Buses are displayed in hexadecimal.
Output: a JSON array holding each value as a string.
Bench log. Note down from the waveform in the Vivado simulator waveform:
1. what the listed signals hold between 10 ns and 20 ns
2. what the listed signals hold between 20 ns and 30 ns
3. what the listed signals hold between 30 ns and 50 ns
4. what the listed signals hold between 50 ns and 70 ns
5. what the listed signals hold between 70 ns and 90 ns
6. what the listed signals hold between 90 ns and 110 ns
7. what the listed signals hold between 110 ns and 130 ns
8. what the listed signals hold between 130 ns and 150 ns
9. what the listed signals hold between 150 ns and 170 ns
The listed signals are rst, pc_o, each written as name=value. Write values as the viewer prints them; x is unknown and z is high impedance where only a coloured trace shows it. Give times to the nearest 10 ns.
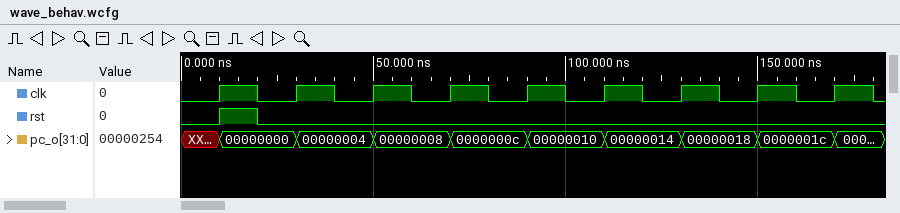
["rst=1, pc_o=00000000", "rst=0, pc_o=00000000", "rst=0, pc_o=00000004", "rst=0, pc_o=00000008", "rst=0, pc_o=0000000c", "rst=0, pc_o=00000010", "rst=0, pc_o=00000014", "rst=0, pc_o=00000018", "rst=0, pc_o=0000001c"]
